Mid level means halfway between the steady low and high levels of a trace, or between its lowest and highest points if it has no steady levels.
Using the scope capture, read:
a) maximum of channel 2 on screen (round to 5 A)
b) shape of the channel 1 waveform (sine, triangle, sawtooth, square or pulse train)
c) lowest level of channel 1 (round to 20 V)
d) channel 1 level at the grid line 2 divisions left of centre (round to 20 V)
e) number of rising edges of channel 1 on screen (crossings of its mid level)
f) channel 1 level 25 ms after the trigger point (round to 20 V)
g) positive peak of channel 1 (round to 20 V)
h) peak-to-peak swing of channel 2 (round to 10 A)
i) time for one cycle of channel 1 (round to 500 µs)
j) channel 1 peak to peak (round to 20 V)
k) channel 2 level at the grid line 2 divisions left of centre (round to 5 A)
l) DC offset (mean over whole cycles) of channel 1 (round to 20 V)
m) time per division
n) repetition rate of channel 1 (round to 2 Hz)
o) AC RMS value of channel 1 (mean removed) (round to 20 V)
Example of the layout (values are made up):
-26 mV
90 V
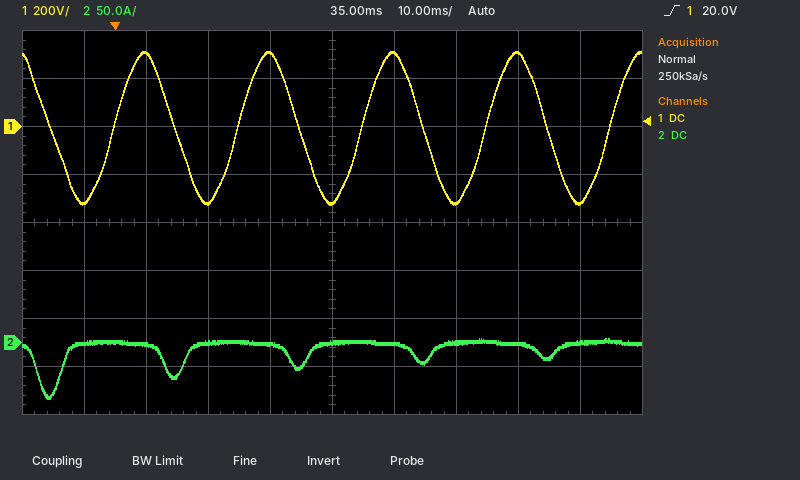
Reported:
5 A
sine
-320 V
-320 V
5
300 V
320 V
60 A
20.0 ms
640 V
0 A
0 V
10 ms
50 Hz
220 V
